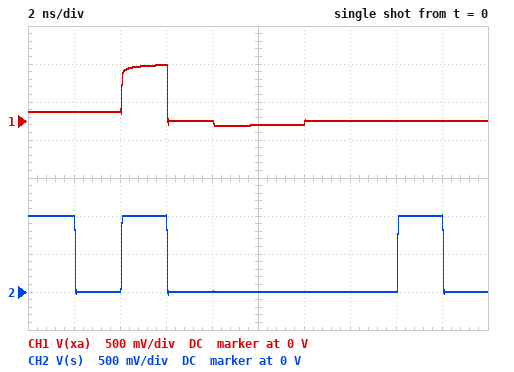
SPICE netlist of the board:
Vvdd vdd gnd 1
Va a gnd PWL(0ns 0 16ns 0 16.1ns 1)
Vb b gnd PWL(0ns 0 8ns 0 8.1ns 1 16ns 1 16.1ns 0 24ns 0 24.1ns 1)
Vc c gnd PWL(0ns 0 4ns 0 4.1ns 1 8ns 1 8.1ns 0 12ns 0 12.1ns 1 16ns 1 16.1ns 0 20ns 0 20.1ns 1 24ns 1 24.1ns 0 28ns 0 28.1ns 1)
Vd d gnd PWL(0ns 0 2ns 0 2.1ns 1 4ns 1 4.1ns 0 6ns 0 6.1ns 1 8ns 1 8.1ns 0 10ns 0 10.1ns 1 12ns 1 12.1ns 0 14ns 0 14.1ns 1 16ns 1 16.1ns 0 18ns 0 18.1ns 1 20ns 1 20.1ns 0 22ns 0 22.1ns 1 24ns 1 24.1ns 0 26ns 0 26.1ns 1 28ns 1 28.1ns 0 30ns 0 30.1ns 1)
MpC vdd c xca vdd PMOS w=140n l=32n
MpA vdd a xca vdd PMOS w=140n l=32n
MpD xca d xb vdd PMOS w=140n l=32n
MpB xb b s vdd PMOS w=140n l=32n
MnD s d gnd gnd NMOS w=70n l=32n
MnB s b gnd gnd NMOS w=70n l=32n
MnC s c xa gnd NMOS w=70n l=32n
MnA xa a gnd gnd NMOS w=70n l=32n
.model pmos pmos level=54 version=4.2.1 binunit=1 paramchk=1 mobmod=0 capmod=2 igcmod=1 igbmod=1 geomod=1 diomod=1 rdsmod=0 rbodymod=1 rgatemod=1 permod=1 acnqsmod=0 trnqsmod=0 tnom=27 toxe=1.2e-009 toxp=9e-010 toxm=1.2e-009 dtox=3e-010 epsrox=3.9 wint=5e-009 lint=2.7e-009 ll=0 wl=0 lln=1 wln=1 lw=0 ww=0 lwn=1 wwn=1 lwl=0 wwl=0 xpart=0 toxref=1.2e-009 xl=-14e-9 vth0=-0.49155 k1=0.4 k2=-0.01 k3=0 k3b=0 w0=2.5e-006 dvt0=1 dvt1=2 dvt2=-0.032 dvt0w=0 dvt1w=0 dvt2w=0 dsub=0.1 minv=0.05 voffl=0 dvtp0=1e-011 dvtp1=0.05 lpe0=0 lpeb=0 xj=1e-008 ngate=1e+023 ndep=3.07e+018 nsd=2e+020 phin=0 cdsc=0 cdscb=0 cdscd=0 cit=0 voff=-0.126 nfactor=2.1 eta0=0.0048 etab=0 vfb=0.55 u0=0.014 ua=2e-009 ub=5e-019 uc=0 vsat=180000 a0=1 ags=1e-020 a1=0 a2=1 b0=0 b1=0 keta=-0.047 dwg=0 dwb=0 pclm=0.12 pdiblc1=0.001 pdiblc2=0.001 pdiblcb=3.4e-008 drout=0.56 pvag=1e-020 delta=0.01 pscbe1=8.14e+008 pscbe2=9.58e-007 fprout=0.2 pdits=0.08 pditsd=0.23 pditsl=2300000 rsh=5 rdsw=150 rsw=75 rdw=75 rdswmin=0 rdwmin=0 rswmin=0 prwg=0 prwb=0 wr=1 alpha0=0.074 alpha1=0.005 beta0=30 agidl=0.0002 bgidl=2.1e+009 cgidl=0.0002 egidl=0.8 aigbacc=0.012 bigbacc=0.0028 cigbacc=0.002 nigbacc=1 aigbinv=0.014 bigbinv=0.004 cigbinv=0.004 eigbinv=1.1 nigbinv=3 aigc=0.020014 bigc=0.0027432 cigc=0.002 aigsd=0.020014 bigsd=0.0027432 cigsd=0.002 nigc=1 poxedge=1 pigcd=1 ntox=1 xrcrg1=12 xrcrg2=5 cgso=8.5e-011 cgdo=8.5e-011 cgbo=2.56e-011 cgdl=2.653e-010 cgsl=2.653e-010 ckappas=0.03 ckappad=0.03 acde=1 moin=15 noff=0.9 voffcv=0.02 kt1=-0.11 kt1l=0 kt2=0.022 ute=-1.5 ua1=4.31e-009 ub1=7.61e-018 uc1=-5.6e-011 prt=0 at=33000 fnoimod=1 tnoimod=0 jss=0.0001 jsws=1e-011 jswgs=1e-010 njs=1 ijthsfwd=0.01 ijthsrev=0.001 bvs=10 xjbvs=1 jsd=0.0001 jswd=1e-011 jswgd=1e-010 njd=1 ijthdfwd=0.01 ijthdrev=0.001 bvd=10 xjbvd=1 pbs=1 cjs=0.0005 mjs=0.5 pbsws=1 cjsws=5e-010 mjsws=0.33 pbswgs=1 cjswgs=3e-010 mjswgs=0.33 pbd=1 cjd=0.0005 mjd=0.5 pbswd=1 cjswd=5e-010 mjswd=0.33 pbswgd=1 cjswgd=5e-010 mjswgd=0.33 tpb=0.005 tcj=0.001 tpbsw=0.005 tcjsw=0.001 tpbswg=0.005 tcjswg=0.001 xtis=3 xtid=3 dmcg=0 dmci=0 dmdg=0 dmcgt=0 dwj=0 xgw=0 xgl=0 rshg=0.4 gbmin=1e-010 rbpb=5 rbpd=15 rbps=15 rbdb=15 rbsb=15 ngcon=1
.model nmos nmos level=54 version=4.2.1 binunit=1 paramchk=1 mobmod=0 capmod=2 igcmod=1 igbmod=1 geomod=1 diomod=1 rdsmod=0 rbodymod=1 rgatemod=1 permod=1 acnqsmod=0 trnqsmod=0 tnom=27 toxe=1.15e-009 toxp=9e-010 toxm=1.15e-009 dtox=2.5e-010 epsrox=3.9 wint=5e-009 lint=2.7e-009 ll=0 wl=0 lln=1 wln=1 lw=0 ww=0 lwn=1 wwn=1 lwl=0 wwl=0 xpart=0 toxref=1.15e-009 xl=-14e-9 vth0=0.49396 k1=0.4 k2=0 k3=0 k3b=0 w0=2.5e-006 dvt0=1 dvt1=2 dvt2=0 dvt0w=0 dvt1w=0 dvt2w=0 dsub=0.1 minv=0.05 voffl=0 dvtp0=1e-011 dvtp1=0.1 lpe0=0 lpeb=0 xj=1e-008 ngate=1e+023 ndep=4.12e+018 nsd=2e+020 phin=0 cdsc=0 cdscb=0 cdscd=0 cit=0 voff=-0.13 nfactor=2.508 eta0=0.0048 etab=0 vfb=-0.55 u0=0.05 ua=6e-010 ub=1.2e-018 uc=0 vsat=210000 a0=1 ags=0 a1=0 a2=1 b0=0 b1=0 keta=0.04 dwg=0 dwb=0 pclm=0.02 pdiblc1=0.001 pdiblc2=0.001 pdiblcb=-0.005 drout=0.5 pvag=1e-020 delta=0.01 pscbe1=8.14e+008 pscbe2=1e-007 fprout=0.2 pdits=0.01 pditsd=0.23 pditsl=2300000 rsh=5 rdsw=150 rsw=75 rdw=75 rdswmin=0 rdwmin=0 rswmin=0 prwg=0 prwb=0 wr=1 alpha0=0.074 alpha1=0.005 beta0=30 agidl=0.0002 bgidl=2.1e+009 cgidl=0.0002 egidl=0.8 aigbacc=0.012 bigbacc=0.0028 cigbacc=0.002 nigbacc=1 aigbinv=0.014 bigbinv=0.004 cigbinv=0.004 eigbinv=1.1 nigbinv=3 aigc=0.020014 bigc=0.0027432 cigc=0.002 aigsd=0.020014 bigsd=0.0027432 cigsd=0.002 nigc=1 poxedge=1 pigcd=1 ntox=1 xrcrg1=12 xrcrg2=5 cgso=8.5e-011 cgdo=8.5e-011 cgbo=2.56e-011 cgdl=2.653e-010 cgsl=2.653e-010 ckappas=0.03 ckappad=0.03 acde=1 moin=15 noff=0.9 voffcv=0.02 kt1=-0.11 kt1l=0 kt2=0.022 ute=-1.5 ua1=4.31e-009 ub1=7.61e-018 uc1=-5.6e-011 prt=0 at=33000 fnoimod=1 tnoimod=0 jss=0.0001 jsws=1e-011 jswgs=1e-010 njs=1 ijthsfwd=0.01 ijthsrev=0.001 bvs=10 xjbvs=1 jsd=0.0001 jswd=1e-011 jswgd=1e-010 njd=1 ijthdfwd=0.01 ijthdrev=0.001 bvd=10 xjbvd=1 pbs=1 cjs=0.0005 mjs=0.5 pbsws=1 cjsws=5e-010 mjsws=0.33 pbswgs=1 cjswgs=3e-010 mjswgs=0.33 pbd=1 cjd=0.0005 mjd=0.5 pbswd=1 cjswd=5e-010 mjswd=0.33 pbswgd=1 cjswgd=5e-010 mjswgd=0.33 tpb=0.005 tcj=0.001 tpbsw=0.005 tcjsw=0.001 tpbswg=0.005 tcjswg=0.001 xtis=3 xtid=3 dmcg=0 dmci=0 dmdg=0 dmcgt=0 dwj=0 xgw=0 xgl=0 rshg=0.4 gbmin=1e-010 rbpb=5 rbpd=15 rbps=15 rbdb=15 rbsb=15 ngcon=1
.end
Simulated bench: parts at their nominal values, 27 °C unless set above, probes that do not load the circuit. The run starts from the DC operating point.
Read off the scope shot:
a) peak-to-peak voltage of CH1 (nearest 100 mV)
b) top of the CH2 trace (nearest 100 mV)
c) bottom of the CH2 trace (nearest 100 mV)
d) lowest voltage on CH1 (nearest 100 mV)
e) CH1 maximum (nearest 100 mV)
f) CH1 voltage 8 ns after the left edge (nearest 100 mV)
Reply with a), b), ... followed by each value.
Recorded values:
a) 800 mV
b) 1.0 V
c) 0 V
d) -100 mV
e) 700 mV
f) 0 V
